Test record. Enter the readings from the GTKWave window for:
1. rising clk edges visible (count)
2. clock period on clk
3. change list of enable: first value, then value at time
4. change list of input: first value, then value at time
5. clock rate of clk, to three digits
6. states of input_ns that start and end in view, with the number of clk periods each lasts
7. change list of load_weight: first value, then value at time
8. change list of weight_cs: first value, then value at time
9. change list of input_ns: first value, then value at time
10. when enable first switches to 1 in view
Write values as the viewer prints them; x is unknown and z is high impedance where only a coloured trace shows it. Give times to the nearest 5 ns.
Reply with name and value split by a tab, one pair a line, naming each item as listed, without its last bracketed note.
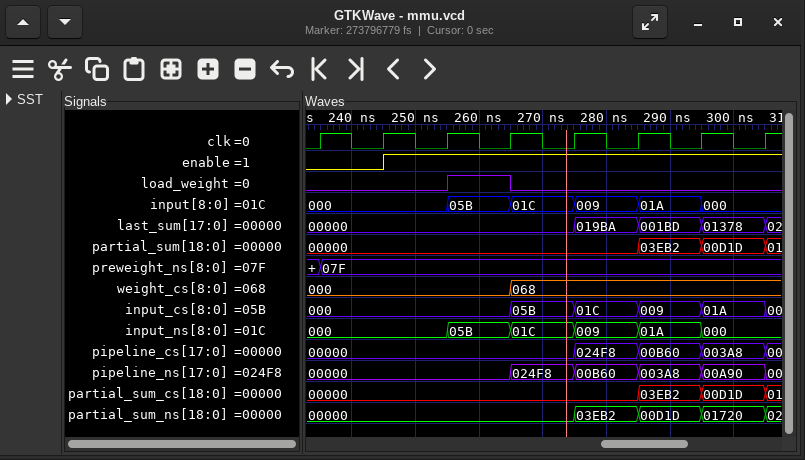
rising clk edges visible	8
clock period on clk	10 ns
change list of enable: first value, then value at time	0, 1 at 245 ns
change list of input: first value, then value at time	000, 05B at 255 ns, 01C at 265 ns, 009 at 275 ns, 01A at 285 ns, 000 at 295 ns
clock rate of clk, to three digits	100 MHz
states of input_ns that start and end in view, with the number of clk periods each lasts	05B: 1, 01C: 1, 009: 1, 01A: 1
change list of load_weight: first value, then value at time	0, 1 at 255 ns, 0 at 265 ns
change list of weight_cs: first value, then value at time	000, 068 at 265 ns
change list of input_ns: first value, then value at time	000, 05B at 255 ns, 01C at 265 ns, 009 at 275 ns, 01A at 285 ns, 000 at 295 ns
when enable first switches to 1 in view	245 ns
